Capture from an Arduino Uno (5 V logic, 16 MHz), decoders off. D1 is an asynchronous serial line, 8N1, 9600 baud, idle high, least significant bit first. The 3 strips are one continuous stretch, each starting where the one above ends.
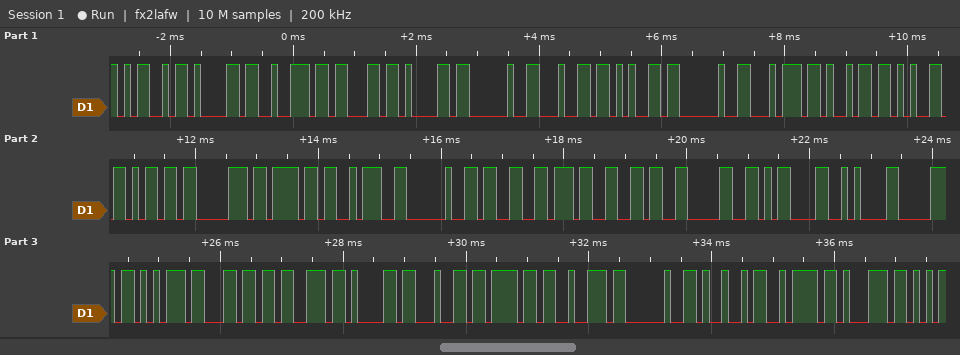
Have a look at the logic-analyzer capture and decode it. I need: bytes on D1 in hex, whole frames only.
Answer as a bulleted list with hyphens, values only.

- 4D 61 72 63 61 20 64 65 20 74 69 65 6D 70 6F 3A 20 33 37 36 30 0D 0A 70 75 6C 73 61 64 6F 72 20 49 7A 71
